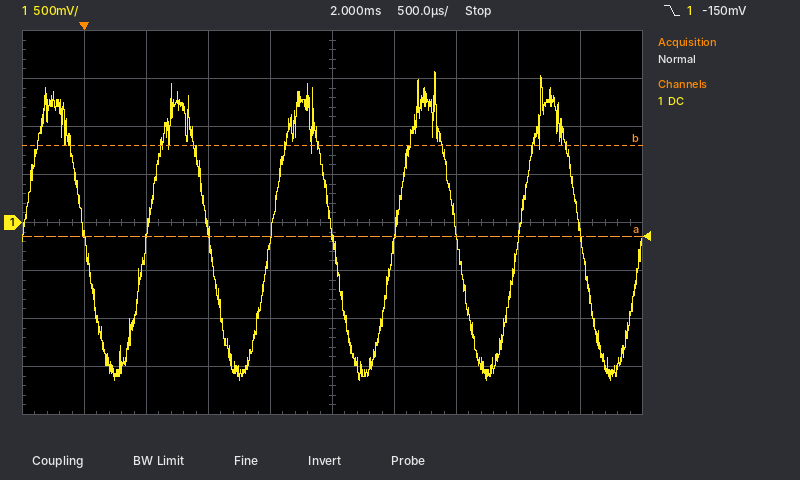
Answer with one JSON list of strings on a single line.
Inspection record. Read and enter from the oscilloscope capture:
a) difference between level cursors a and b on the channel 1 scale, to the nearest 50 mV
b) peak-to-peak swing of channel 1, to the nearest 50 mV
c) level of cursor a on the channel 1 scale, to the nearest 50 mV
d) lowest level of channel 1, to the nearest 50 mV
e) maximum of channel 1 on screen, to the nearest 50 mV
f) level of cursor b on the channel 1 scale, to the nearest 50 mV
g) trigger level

["950 mV", "3.20 V", "-150 mV", "-1.65 V", "1.55 V", "800 mV", "-150 mV"]
